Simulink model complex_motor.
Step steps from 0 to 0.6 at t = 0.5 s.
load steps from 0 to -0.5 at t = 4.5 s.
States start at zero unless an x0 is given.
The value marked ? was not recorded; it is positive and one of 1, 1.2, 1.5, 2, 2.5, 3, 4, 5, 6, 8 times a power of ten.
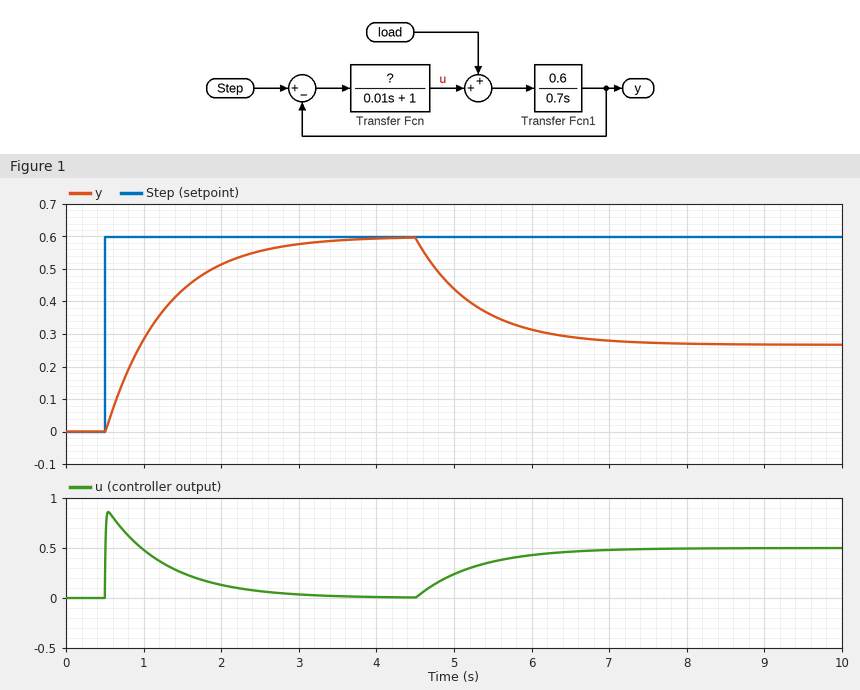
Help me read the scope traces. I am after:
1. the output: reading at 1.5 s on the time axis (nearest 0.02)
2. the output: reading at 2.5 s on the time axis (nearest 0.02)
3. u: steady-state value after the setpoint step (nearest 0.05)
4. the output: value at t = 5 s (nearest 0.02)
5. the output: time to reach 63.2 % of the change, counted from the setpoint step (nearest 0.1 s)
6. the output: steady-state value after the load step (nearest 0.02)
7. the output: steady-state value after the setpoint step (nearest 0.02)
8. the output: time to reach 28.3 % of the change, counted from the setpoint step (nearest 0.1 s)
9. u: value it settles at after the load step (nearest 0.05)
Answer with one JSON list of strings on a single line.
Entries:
["0.44", "0.56", "0.00", "0.44", "0.8 s", "0.26", "0.60", "0.3 s", "0.50"]
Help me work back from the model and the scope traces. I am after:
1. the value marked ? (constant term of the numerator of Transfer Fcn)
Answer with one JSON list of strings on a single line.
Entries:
["1.5"]
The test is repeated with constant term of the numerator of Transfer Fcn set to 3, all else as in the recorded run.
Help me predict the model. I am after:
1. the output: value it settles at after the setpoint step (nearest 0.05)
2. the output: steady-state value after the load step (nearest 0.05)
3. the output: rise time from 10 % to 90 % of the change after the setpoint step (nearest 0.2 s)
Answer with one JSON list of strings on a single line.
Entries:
["0.60", "0.45", "0.8 s"]
